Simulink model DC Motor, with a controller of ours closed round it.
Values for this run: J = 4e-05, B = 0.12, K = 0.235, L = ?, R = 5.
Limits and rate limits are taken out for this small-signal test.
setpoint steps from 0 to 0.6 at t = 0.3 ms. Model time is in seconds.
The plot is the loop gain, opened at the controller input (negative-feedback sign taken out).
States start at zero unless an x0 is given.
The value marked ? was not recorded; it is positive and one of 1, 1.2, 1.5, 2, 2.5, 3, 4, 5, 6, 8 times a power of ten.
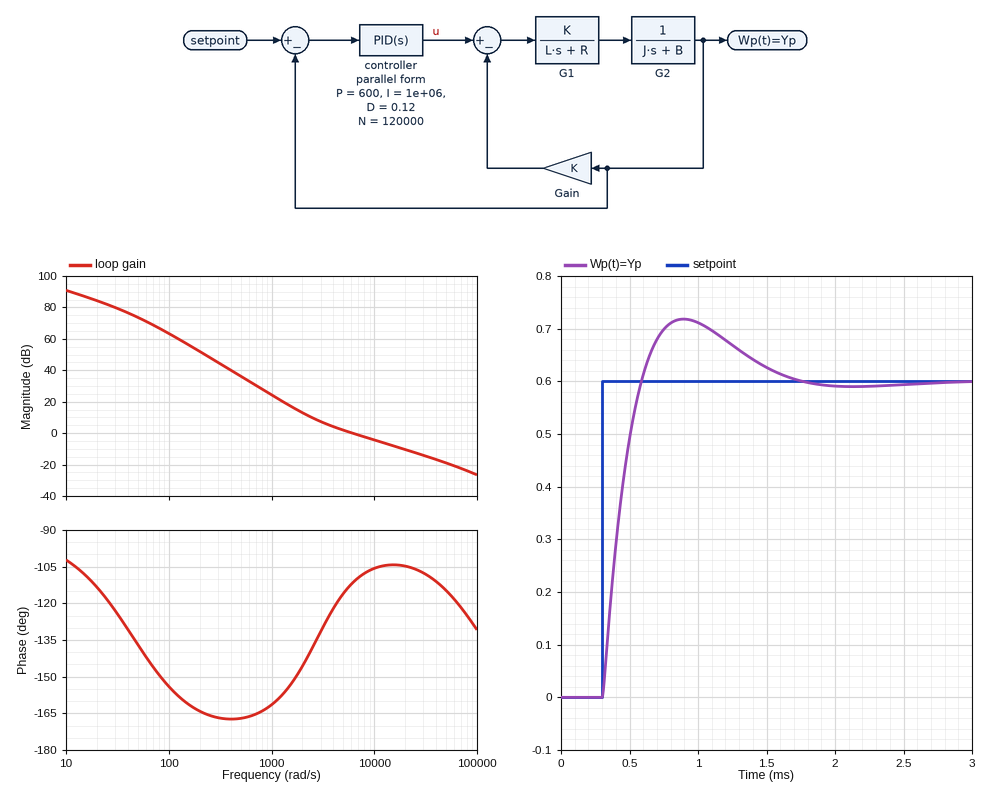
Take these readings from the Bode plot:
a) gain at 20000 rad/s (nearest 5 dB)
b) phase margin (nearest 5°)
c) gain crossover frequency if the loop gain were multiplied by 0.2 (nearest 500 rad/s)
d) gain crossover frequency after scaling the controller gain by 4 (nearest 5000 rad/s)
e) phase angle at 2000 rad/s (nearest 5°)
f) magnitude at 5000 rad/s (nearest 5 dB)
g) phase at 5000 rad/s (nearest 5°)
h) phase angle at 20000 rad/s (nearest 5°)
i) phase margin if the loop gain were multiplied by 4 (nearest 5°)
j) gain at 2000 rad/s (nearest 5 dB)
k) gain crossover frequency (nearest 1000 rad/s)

-10 dB
70°
2000 rad/s
25000 rad/s
-145°
0 dB
-115°
-105°
75°
15 dB
6000 rad/s
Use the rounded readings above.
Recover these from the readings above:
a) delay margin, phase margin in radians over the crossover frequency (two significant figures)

0.00020 s
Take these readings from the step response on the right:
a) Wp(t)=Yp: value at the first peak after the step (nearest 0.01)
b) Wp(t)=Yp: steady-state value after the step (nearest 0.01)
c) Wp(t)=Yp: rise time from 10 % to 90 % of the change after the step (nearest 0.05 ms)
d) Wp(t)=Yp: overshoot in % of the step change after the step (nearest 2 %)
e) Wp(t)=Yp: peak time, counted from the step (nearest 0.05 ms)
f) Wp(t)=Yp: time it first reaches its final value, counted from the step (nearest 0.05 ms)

0.72
0.60
0.20 ms
20 %
0.60 ms
0.30 ms
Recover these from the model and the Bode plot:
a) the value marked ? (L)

0.12
